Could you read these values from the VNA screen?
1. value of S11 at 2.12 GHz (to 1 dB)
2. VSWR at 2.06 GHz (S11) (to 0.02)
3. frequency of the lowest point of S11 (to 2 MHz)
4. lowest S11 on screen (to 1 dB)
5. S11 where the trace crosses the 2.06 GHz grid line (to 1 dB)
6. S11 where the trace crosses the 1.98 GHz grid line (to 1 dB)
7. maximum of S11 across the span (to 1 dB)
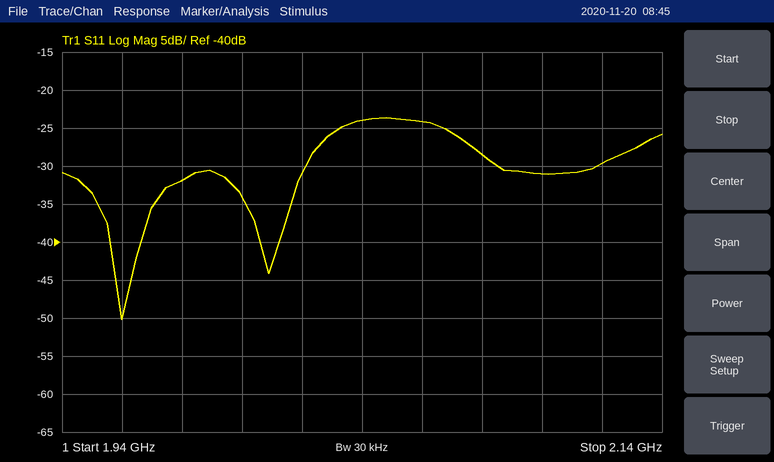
-30 dB
1.14
1.960 GHz
-50 dB
-24 dB
-32 dB
-24 dB
